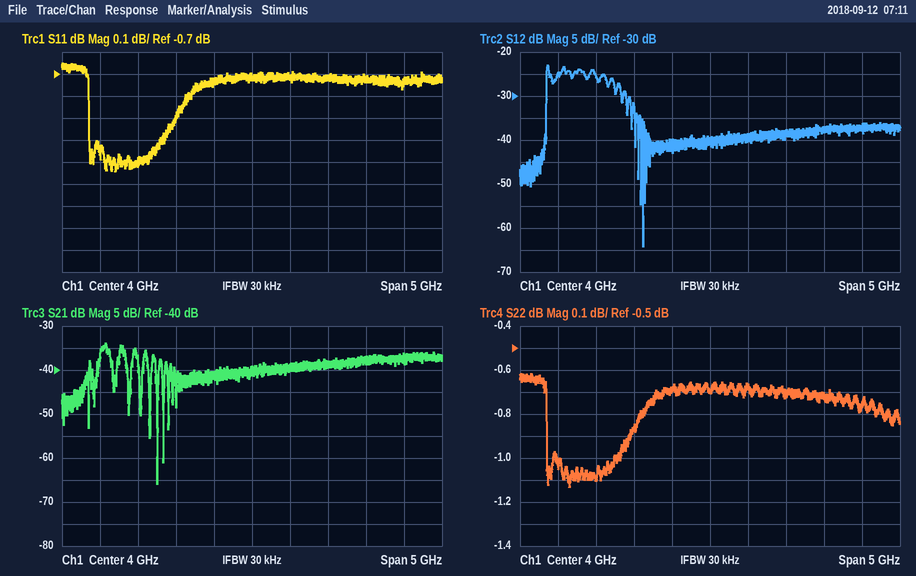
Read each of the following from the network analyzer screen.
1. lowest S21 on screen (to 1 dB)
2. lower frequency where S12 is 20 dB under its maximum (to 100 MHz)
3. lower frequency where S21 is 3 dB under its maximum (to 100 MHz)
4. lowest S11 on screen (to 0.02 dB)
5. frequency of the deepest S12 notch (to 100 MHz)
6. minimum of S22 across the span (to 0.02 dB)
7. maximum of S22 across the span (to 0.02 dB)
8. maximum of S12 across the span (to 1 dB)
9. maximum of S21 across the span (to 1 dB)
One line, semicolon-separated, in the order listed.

-66 dB; 1.8 GHz; 2.0 GHz; -1.14 dB; 3.1 GHz; -1.14 dB; -0.62 dB; -23 dB; -34 dB
